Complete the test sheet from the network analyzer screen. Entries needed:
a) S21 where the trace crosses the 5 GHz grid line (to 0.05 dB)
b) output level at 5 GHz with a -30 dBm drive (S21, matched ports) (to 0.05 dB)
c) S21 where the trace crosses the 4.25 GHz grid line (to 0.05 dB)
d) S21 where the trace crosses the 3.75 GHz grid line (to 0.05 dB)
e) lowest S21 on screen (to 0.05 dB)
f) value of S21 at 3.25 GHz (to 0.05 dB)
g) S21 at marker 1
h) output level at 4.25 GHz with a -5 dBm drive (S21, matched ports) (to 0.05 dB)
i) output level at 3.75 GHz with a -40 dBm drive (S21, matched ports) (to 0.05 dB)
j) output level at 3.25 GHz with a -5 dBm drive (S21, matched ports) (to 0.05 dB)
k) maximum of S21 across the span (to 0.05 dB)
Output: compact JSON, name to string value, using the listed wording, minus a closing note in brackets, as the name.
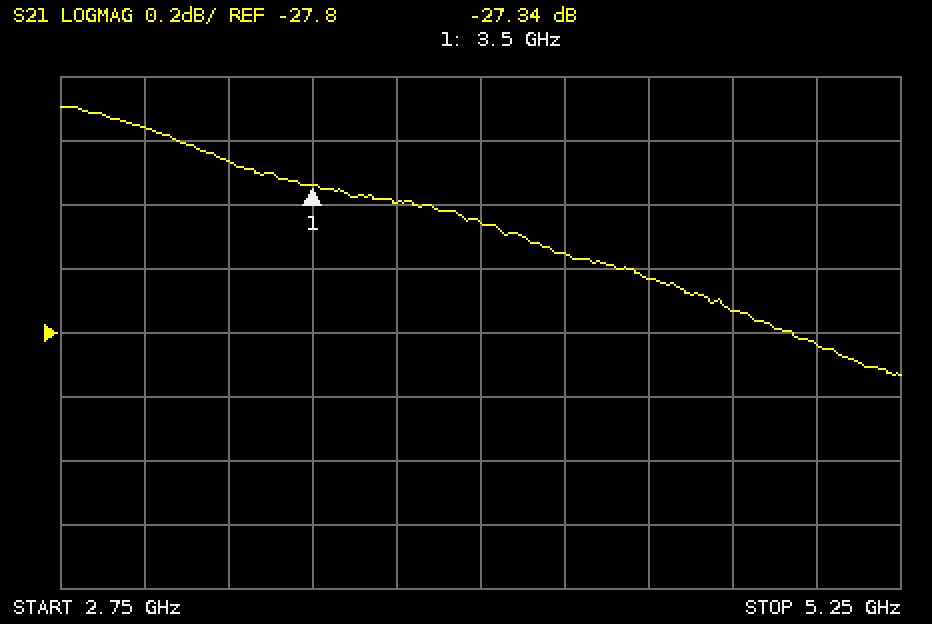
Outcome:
{"S21 where the trace crosses the 5 GHz grid line": "-27.85 dB", "output level at 5 GHz with a -30 dBm drive (S21, matched ports)": "-57.85 dBm", "S21 where the trace crosses the 4.25 GHz grid line": "-27.55 dB", "S21 where the trace crosses the 3.75 GHz grid line": "-27.40 dB", "lowest S21 on screen": "-27.95 dB", "value of S21 at 3.25 GHz": "-27.25 dB", "S21 at marker 1": "-27.34 dB", "output level at 4.25 GHz with a -5 dBm drive (S21, matched ports)": "-32.55 dBm", "output level at 3.75 GHz with a -40 dBm drive (S21, matched ports)": "-67.40 dBm", "output level at 3.25 GHz with a -5 dBm drive (S21, matched ports)": "-32.25 dBm", "maximum of S21 across the span": "-27.10 dB"}
